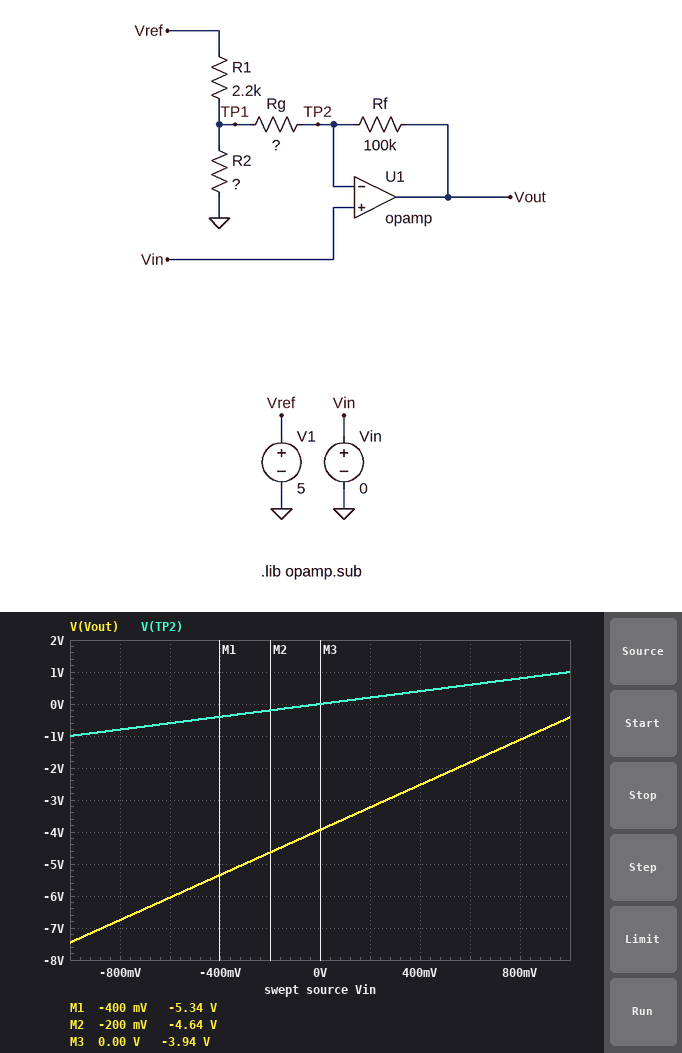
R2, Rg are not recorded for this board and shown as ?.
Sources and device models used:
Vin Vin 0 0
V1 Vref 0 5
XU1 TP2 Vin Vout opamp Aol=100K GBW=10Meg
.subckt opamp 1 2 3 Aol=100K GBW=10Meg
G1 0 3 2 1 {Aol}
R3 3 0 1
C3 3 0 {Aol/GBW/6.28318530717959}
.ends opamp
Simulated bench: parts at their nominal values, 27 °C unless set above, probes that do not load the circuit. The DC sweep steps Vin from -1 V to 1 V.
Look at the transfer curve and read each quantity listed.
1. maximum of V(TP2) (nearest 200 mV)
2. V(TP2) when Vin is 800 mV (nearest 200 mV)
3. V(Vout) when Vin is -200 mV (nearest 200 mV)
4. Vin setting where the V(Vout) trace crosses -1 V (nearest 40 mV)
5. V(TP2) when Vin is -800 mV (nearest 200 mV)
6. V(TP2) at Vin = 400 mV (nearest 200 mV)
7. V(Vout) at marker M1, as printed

1.0 V
800 mV
-4.6 V
840 mV
-800 mV
400 mV
-5.34 V
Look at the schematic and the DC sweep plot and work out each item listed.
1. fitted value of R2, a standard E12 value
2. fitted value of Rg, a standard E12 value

1 kΩ
39 kΩ
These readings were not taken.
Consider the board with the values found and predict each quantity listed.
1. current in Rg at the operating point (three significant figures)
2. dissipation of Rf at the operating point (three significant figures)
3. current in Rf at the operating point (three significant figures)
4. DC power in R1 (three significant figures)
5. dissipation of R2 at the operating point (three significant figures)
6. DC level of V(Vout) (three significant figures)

39.4 µA
155 µW
39.4 µA
5.46 mW
2.36 mW
-3.94 V
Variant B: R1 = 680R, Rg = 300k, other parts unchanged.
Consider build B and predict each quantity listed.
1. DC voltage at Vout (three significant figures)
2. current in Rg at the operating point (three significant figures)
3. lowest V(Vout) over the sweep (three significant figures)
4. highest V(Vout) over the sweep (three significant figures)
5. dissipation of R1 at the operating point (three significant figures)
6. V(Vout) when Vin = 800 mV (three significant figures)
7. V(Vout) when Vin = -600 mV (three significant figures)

-991 mV
9.91 µA
-2.32 V
342 mV
6.05 mW
75.6 mV
-1.79 V
